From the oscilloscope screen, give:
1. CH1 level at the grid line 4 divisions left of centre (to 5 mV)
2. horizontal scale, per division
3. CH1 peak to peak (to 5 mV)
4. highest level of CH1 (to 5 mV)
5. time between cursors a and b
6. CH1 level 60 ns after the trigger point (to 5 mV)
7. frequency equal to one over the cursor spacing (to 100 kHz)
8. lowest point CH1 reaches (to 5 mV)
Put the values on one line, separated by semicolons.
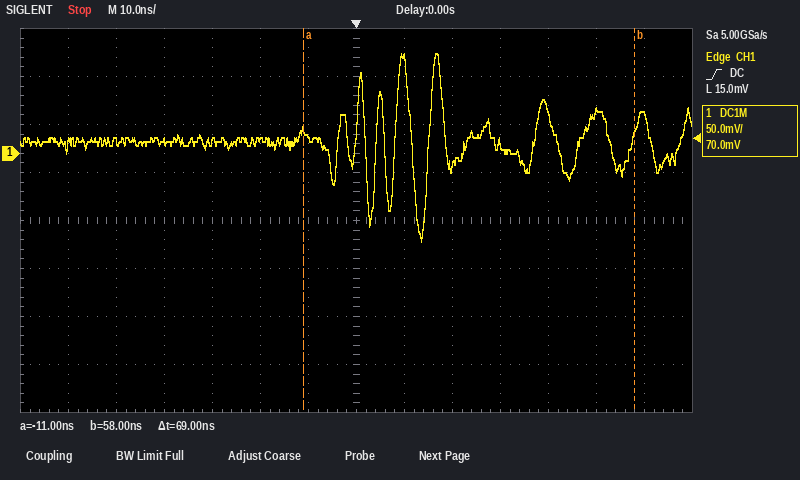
10 mV; 10 ns; 195 mV; 105 mV; 69 ns; 40 mV; 14.5 MHz; -90 mV
